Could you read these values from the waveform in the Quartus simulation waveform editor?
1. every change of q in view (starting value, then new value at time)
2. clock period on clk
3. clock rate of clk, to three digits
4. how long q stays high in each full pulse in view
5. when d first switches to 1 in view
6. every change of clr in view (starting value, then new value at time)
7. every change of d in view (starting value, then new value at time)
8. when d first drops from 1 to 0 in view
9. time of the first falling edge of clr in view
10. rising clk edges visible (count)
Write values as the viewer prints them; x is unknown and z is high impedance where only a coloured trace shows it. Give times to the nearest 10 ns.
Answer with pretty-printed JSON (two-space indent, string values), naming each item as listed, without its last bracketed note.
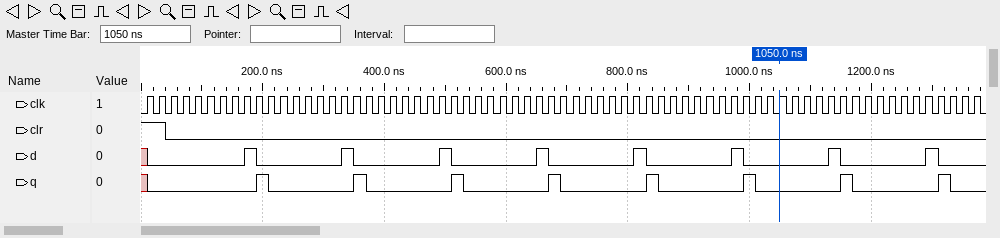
{
  "every change of q in view": "x, 0 at 10 ns, 1 at 190 ns, 0 at 210 ns, 1 at 350 ns, 0 at 370 ns, 1 at 510 ns, 0 at 530 ns, 1 at 670 ns, 0 at 690 ns, 1 at 830 ns, 0 at 850 ns, 1 at 990 ns, 0 at 1010 ns, 1 at 1150 ns, 0 at 1170 ns, 1 at 1310 ns, 0 at 1330 ns",
  "clock period on clk": "20 ns",
  "clock rate of clk, to three digits": "50.0 MHz",
  "how long q stays high in each full pulse in view": "20 ns, 20 ns, 20 ns, 20 ns, 20 ns, 20 ns, 20 ns, 20 ns",
  "when d first switches to 1 in view": "170 ns",
  "every change of clr in view": "1, 0 at 40 ns",
  "every change of d in view": "x, 0 at 10 ns, 1 at 170 ns, 0 at 190 ns, 1 at 330 ns, 0 at 350 ns, 1 at 490 ns, 0 at 510 ns, 1 at 650 ns, 0 at 670 ns, 1 at 810 ns, 0 at 830 ns, 1 at 970 ns, 0 at 990 ns, 1 at 1130 ns, 0 at 1150 ns, 1 at 1290 ns, 0 at 1310 ns",
  "when d first drops from 1 to 0 in view": "190 ns",
  "time of the first falling edge of clr in view": "40 ns",
  "rising clk edges visible": "69"
}
